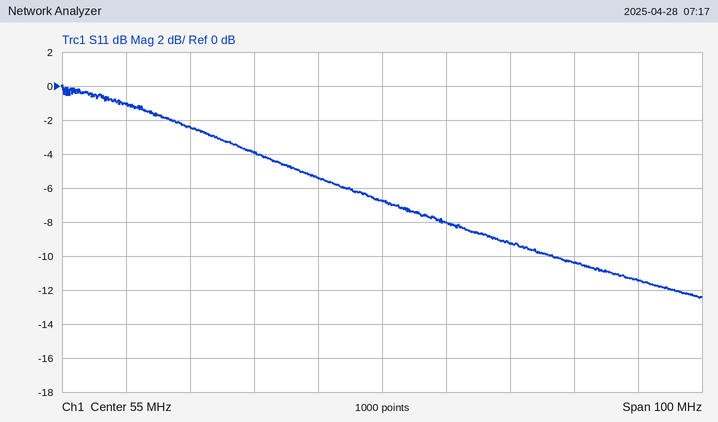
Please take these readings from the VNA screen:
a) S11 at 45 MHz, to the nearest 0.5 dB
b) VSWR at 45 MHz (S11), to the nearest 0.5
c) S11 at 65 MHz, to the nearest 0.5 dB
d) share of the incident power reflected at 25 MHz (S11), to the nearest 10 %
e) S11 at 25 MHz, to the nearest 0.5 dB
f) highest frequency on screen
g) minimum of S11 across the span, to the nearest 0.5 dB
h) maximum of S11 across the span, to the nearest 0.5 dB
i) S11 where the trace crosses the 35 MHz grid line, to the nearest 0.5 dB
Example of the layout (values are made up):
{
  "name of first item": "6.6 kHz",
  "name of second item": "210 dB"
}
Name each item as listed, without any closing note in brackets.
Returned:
{
  "S11 at 45 MHz, to the nearest 0.5 dB": "-5.5 dB",
  "VSWR at 45 MHz (S11), to the nearest 0.5": "3.5",
  "S11 at 65 MHz, to the nearest 0.5 dB": "-8.0 dB",
  "share of the incident power reflected at 25 MHz (S11), to the nearest 10 %": "60 %",
  "S11 at 25 MHz, to the nearest 0.5 dB": "-2.5 dB",
  "highest frequency on screen": "105 MHz",
  "minimum of S11 across the span, to the nearest 0.5 dB": "-12.5 dB",
  "maximum of S11 across the span, to the nearest 0.5 dB": "0.0 dB",
  "S11 where the trace crosses the 35 MHz grid line, to the nearest 0.5 dB": "-4.0 dB"
}
